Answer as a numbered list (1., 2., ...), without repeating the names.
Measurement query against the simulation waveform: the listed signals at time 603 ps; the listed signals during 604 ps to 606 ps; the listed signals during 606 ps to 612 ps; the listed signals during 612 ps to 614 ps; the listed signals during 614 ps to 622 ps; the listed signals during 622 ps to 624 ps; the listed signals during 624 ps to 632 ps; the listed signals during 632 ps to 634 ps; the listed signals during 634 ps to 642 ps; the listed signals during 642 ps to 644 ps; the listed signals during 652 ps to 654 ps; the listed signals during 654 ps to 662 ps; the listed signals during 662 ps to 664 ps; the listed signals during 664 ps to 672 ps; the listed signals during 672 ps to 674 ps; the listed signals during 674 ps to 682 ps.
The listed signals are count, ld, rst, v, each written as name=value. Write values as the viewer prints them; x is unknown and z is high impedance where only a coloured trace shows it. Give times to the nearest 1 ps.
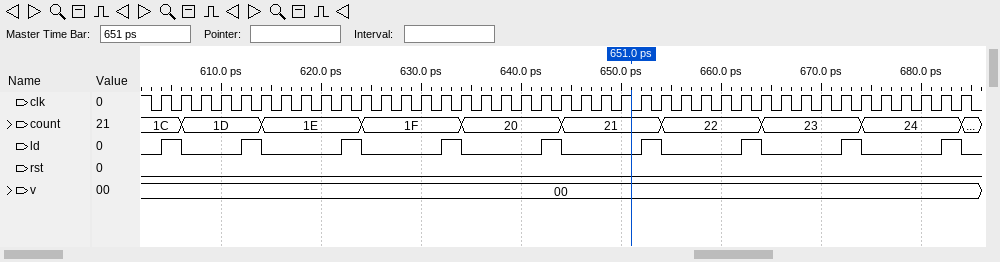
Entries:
1. count=1C, ld=0, rst=0, v=00
2. count=1C, ld=1, rst=0, v=00
3. count=1D, ld=0, rst=0, v=00
4. count=1D, ld=1, rst=0, v=00
5. count=1E, ld=0, rst=0, v=00
6. count=1E, ld=1, rst=0, v=00
7. count=1F, ld=0, rst=0, v=00
8. count=1F, ld=1, rst=0, v=00
9. count=20, ld=0, rst=0, v=00
10. count=20, ld=1, rst=0, v=00
11. count=21, ld=1, rst=0, v=00
12. count=22, ld=0, rst=0, v=00
13. count=22, ld=1, rst=0, v=00
14. count=23, ld=0, rst=0, v=00
15. count=23, ld=1, rst=0, v=00
16. count=24, ld=0, rst=0, v=00
